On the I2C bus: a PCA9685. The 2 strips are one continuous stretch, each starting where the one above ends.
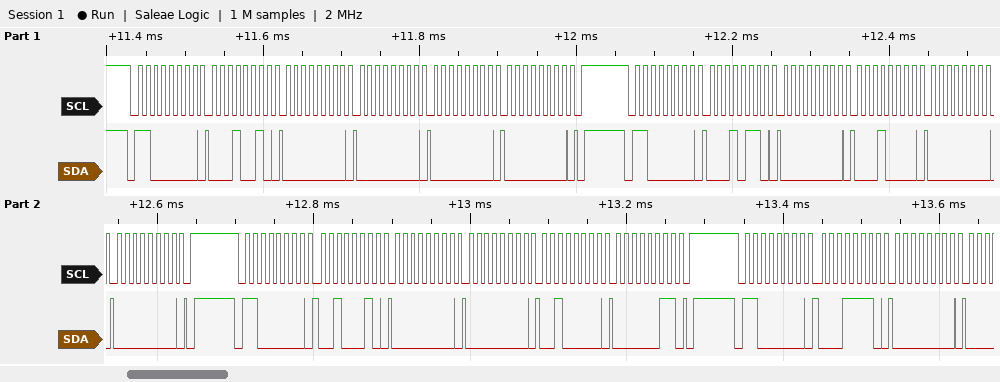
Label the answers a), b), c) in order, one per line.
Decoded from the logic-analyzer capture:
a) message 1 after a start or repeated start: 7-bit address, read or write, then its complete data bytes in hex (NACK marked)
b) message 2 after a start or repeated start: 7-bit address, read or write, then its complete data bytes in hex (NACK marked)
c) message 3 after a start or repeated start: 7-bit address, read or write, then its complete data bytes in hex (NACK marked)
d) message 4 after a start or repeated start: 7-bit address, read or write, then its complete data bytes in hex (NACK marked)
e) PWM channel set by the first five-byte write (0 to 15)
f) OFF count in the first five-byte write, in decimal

a) 0x60 write: 12 00 00 00 00
b) 0x60 write: 16 00 10 00 00
c) 0x60 write: 22 00 00 20 03
d) 0x60 write: 1E 00
e) 3
f) 0
